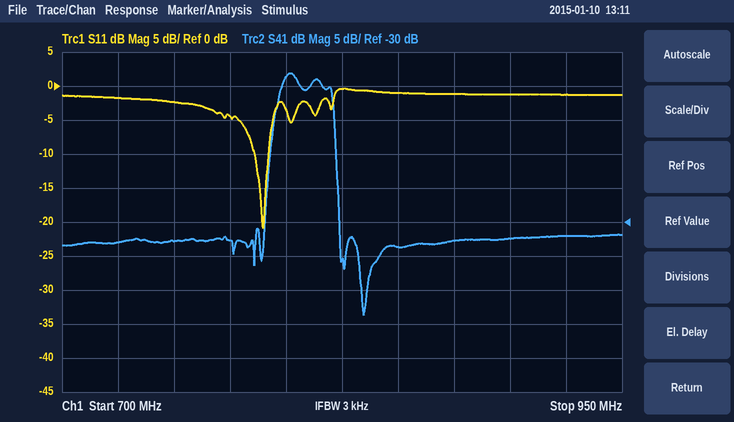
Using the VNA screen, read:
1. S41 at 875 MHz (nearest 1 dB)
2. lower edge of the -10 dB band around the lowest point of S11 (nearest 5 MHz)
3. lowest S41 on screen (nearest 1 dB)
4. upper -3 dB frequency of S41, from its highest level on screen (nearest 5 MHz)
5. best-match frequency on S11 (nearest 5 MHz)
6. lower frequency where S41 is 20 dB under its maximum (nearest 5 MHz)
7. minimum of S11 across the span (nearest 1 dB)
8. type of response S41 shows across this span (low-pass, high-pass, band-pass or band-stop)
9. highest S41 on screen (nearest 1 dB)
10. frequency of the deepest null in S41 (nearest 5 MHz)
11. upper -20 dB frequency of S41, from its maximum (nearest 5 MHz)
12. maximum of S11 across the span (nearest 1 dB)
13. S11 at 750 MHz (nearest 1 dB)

-33 dB
785 MHz
-44 dB
820 MHz
790 MHz
790 MHz
-21 dB
band-pass
-8 dB
835 MHz
825 MHz
0 dB
-2 dB
